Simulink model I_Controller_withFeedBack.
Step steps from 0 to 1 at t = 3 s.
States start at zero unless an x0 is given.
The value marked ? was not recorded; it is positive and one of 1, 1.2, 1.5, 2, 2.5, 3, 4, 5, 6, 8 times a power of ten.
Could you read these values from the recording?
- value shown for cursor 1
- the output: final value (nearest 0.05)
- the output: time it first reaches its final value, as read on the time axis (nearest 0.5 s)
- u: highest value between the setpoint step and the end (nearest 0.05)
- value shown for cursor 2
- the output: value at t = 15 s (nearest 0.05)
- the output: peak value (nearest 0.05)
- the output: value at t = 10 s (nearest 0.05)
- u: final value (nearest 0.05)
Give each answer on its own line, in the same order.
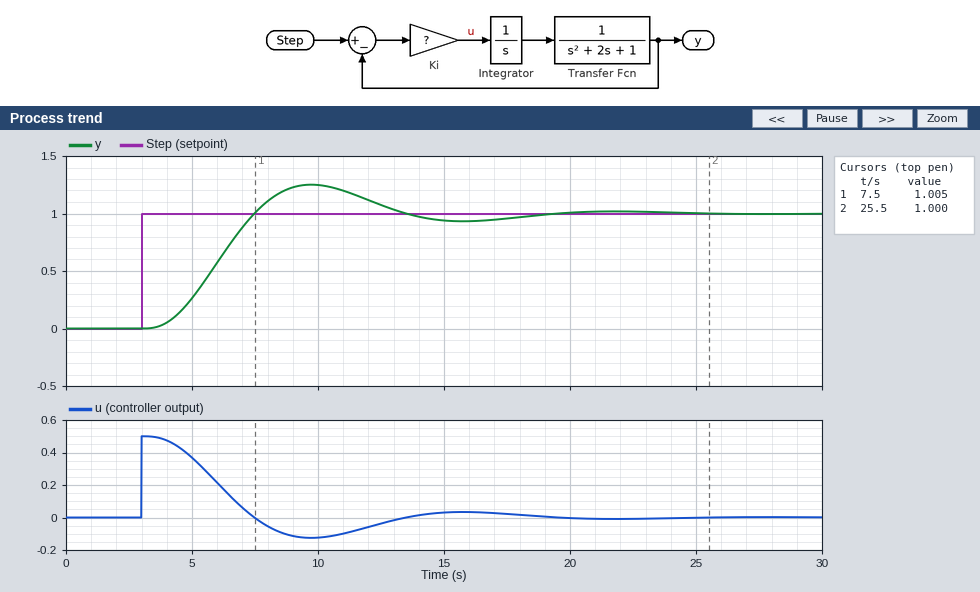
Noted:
1.005
1.00
7.5 s
0.50
1.000
0.95
1.25
1.25
0.00
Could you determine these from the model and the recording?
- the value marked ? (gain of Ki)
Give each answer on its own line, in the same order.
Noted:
0.5
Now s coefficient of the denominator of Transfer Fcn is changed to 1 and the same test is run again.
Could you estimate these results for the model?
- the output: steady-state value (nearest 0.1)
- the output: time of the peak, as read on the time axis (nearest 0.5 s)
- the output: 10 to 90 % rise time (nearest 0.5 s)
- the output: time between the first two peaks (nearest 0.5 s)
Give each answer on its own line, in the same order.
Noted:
1.0
8.0 s
2.0 s
7.0 s
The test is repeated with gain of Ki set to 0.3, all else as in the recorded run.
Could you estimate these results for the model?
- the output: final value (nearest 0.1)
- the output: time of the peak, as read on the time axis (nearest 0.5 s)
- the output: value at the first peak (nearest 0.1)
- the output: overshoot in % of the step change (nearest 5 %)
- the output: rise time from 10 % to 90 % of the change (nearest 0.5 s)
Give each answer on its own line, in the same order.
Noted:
1.0
12.5 s
1.1
10 %
4.5 s
